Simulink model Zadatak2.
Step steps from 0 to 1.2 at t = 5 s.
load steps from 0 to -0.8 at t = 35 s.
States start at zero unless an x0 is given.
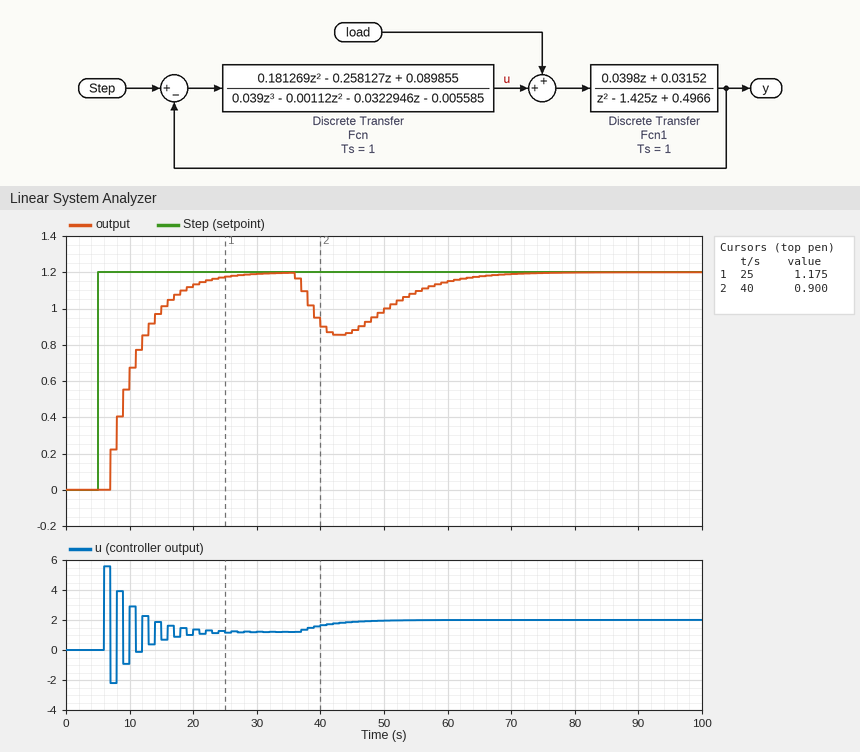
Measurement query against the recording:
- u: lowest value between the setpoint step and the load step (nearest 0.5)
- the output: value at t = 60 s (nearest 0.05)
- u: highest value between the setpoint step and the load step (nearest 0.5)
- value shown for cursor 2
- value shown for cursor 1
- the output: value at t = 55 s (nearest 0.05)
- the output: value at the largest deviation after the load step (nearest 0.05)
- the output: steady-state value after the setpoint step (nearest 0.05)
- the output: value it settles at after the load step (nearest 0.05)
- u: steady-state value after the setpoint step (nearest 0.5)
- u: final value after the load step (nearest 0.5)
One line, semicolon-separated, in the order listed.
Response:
-2.0; 1.15; 5.5; 0.900; 1.175; 1.10; 0.85; 1.20; 1.20; 1.0; 2.0
